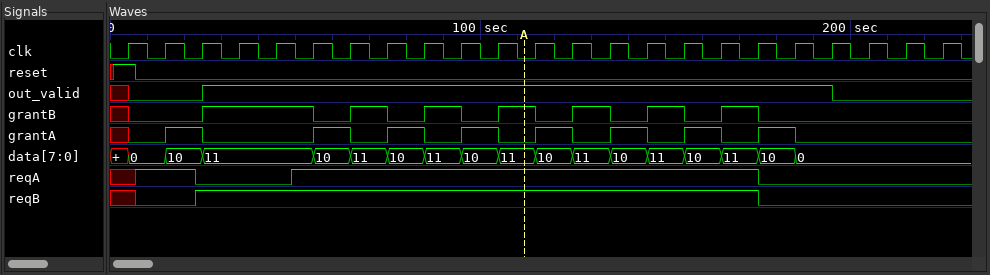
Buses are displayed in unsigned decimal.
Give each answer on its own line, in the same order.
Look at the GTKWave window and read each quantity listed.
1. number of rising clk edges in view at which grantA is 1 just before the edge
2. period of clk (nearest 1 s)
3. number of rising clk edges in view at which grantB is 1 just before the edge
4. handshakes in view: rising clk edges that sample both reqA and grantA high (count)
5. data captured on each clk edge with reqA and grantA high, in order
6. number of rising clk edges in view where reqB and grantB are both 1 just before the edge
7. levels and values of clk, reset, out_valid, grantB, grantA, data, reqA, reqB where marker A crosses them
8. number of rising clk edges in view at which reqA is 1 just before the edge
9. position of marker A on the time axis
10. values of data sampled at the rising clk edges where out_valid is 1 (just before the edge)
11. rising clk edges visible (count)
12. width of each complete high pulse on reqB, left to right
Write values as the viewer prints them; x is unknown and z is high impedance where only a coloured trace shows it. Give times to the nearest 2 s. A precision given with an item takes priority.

8
10 s
9
6
10, 10, 10, 10, 10, 10
9
clk=0, reset=0, out_valid=1, grantB=1, grantA=0, data=11, reqA=1, reqB=1
14
112 s
11, 11, 11, 10, 11, 10, 11, 10, 11, 10, 11, 10, 11, 10, 11, 10, 0
23
152 s
